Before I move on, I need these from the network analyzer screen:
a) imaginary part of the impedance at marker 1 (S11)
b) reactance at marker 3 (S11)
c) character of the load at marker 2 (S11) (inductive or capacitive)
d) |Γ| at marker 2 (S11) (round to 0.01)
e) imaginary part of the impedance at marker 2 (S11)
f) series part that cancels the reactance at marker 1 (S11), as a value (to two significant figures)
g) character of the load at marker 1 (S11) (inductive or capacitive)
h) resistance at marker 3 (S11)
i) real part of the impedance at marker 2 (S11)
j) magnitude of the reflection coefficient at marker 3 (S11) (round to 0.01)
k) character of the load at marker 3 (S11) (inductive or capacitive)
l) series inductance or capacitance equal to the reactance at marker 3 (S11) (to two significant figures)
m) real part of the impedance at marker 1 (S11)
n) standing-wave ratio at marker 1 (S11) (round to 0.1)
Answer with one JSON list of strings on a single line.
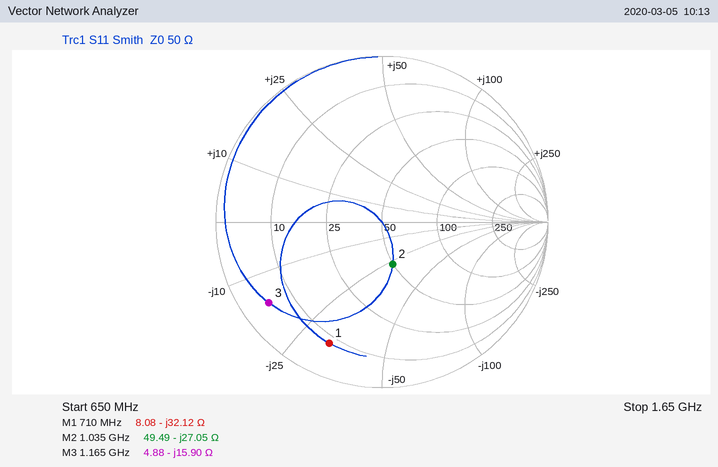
["-32.12 Ω", "-15.90 Ω", "capacitive", "0.26", "-27.05 Ω", "7.2 nH", "capacitive", "4.88 Ω", "49.49 Ω", "0.84", "capacitive", "8.6 pF", "8.08 Ω", "8.8"]
